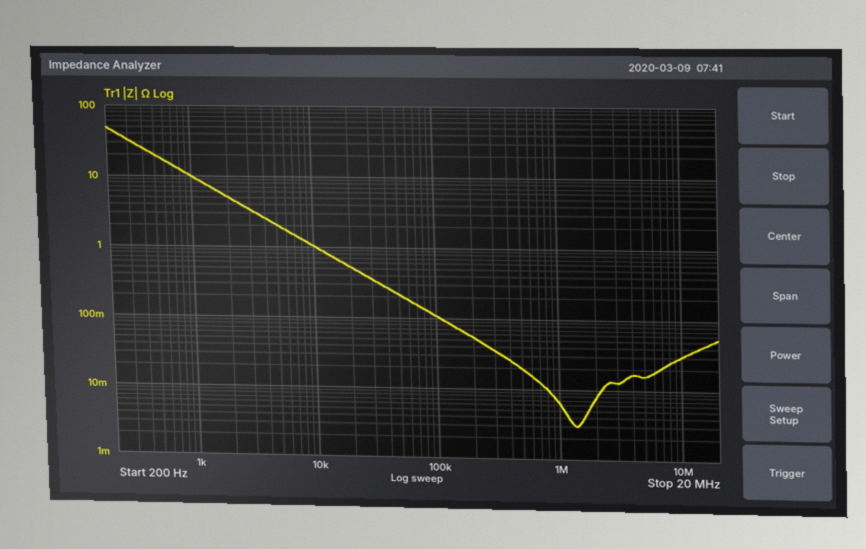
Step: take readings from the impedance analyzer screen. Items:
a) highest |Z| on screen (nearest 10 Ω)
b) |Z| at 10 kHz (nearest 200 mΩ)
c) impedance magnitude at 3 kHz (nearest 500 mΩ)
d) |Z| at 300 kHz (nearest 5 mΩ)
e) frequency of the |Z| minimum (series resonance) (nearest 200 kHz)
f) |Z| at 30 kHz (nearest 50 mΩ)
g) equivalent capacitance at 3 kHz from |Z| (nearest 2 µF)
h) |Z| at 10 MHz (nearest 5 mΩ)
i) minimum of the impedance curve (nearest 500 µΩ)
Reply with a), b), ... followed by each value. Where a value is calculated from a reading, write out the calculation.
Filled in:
a) 50 Ω
b) 1.0 Ω
c) 3.5 Ω
d) 35 mΩ
e) 1.4 MHz
f) 350 mΩ
g) C = 1/(2π × 3 kHz × 3.5 Ω) ≈ 15.2 µF, so 16 µF to the nearest 2 µF
h) 30 mΩ
i) 3.0 mΩ
